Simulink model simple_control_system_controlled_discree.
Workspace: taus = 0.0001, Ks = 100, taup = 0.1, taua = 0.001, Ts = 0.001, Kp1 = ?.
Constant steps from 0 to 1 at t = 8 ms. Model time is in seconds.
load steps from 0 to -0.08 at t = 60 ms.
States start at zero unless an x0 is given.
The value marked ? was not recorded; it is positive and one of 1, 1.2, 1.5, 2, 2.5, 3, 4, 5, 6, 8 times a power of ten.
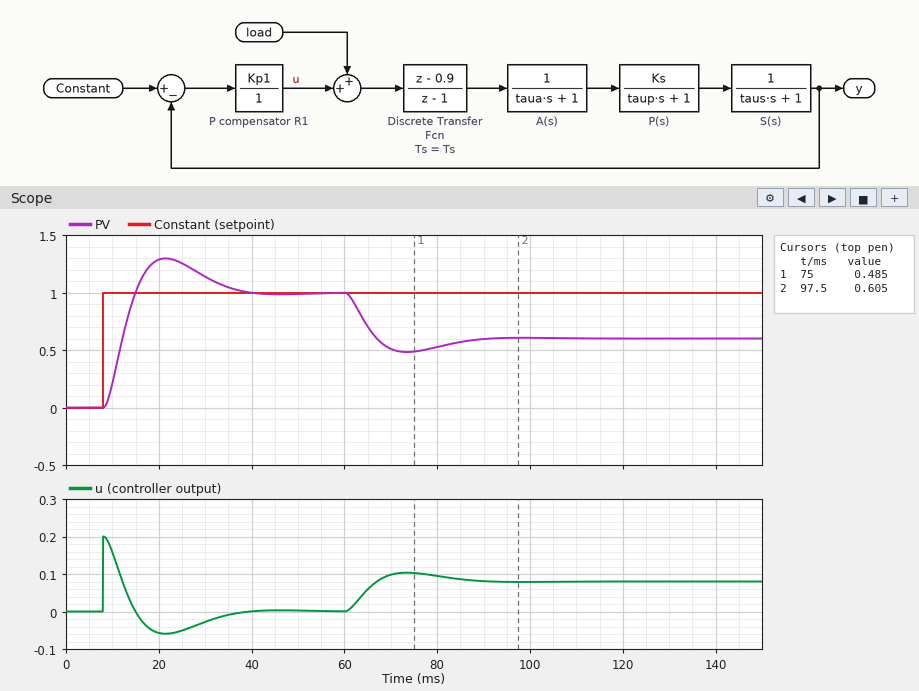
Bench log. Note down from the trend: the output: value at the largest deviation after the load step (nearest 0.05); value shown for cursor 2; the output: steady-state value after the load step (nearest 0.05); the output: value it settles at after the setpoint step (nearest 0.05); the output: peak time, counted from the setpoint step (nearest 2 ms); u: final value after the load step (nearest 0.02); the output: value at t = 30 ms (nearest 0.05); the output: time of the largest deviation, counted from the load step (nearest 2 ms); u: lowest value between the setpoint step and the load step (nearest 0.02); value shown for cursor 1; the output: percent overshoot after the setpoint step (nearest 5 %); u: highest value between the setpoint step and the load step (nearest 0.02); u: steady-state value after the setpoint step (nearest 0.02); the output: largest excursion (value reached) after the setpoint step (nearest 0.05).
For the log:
0.50
0.605
0.60
1.00
14 ms
0.08
1.15
14 ms
-0.06
0.485
30 %
0.20
0.00
1.30
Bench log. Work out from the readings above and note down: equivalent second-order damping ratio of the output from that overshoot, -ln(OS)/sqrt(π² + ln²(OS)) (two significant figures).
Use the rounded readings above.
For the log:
0.36
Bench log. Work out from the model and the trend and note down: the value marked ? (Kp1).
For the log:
0.2
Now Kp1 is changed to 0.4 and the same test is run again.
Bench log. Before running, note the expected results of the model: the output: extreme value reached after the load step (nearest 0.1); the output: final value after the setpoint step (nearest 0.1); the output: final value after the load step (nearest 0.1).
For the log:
0.7
1.0
0.8
